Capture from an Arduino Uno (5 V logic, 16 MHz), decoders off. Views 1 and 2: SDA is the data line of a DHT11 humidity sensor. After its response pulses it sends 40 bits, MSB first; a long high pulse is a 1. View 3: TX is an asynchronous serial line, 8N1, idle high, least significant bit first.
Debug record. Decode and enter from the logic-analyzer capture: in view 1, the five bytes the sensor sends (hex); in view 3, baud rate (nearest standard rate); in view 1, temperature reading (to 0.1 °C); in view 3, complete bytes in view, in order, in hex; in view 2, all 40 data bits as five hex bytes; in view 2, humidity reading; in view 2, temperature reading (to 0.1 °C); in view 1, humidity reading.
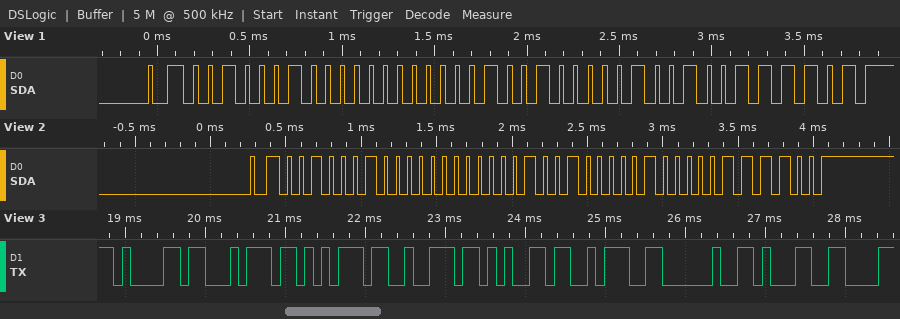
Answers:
22 00 12 09 3D
9600 baud
18.9 °C
0x61 0x74 0x75 0x72 0x65 0x3A 0x20 0x31
22 00 12 08 3C
34 %
18.8 °C
34 %
